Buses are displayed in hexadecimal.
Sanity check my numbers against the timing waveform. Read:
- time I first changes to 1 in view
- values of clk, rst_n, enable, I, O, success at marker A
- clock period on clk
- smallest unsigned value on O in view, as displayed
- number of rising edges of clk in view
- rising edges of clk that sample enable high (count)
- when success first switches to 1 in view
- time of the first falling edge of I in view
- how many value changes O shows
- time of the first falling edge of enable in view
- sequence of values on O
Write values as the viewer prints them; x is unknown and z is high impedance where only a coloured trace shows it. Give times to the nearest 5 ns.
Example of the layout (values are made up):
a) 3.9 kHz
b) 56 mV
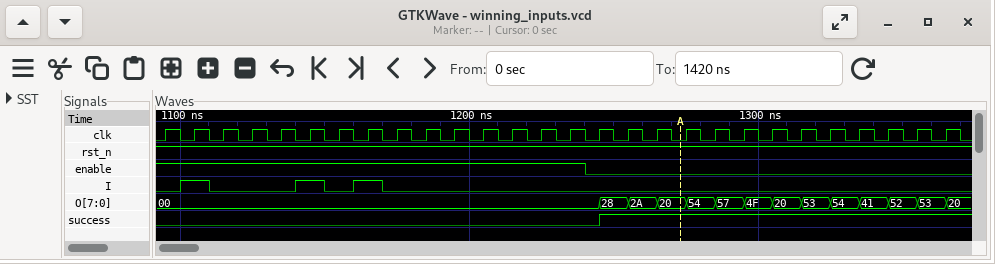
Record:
a) 1100 ns
b) clk=0, rst_n=1, enable=0, I=0, O=20, success=1
c) 10 ns
d) 00
e) 28
f) 15
g) 1245 ns
h) 1110 ns
i) 13
j) 1240 ns
k) 00, 28, 2A, 20, 54, 57, 4F, 20, 53, 54, 41, 52, 53, 20
